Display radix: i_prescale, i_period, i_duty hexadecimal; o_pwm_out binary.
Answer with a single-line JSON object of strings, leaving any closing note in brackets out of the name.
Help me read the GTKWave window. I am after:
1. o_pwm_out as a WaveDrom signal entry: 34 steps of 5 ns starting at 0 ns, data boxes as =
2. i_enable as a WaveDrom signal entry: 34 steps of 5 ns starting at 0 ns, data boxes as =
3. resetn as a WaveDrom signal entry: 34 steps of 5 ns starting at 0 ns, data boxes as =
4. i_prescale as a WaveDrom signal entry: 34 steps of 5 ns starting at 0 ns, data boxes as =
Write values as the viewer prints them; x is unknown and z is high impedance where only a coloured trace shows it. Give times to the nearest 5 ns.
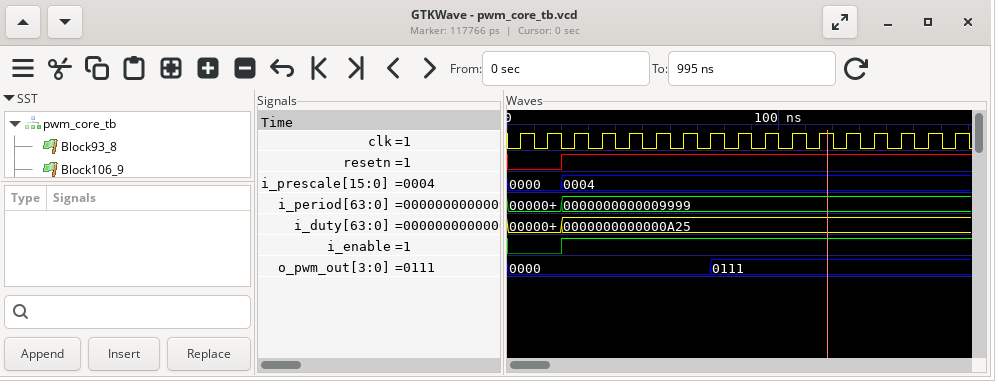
{"o_pwm_out as a WaveDrom signal entry: 34 steps of 5 ns starting at 0 ns, data boxes as =": "{name: 'o_pwm_out', wave: '=..............=..................', data: '0000 0111'}", "i_enable as a WaveDrom signal entry: 34 steps of 5 ns starting at 0 ns, data boxes as =": "{name: 'i_enable', wave: '0...1.............................'}", "resetn as a WaveDrom signal entry: 34 steps of 5 ns starting at 0 ns, data boxes as =": "{name: 'resetn', wave: '0...1.............................'}", "i_prescale as a WaveDrom signal entry: 34 steps of 5 ns starting at 0 ns, data boxes as =": "{name: 'i_prescale', wave: '=...=.............................', data: '0000 0004'}"}
